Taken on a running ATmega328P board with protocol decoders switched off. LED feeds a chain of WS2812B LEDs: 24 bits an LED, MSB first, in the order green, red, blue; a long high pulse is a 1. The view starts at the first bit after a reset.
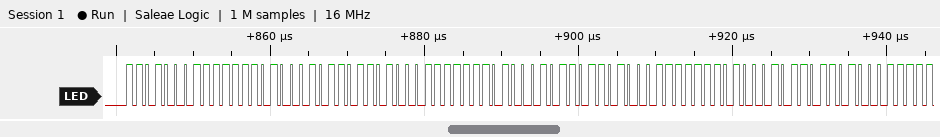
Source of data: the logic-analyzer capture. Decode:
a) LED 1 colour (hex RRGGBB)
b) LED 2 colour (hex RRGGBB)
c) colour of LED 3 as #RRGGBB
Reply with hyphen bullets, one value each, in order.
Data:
- #FDD116
- #FDD116
- #FDD116
